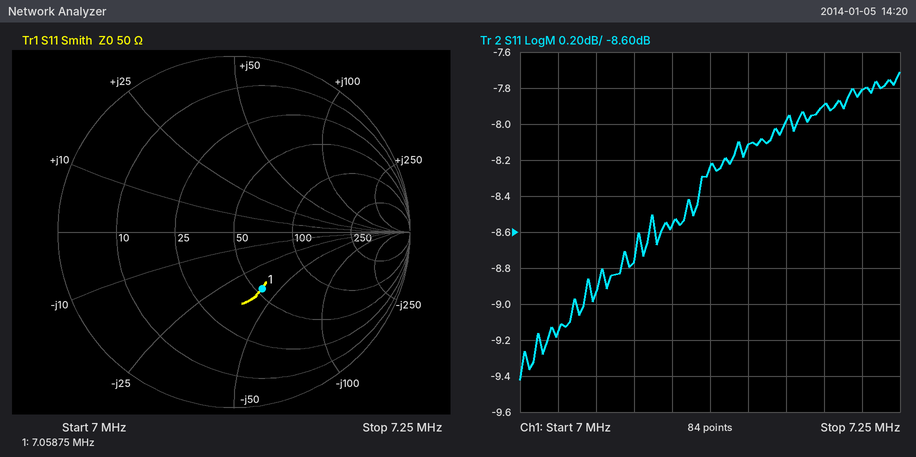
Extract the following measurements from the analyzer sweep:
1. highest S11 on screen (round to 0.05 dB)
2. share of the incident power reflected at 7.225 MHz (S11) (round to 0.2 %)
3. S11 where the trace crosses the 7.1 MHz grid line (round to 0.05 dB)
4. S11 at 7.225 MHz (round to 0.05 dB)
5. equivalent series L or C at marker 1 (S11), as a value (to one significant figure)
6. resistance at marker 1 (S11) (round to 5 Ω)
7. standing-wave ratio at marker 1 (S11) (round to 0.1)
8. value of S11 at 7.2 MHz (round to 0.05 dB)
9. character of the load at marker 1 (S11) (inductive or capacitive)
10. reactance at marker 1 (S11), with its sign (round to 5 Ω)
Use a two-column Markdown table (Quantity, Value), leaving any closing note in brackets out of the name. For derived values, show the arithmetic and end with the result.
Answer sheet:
| Quantity | Value |
|---|---|
| highest S11 on screen | -7.70 dB |
| share of the incident power reflected at 7.225 MHz (S11) | 10^(-7.8/10) ≈ 16.6 % |
| S11 where the trace crosses the 7.1 MHz grid line | -8.55 dB |
| S11 at 7.225 MHz | -7.80 dB |
| equivalent series L or C at marker 1 (S11), as a value | C = 1/(2π × 7.05875 MHz × 40 Ω) ≈ 564 pF, so 600 pF to one significant figure |
| resistance at marker 1 (S11) | 55 Ω |
| standing-wave ratio at marker 1 (S11) | 2.1 |
| value of S11 at 7.2 MHz | -7.90 dB |
| character of the load at marker 1 (S11) | capacitive |
| reactance at marker 1 (S11), with its sign | -40 Ω |
